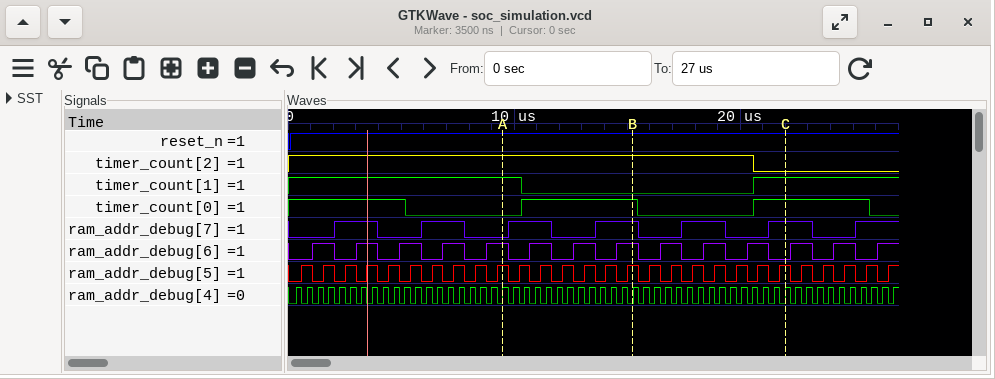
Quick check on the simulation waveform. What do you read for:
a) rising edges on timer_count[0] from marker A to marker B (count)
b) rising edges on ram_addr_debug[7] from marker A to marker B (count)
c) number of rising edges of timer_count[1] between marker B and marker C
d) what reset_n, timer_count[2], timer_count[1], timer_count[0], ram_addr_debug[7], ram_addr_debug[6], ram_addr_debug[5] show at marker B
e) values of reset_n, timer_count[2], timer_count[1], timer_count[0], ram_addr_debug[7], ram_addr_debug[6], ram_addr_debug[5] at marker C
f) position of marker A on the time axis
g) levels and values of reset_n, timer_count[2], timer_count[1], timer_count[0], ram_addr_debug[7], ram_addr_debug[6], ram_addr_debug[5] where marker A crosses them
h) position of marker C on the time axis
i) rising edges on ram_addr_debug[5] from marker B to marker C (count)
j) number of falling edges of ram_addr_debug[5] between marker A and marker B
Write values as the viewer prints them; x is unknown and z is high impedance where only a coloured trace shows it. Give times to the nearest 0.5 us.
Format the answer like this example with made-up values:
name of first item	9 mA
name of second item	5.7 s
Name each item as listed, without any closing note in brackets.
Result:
rising edges on timer_count[0] from marker A to marker B	1
rising edges on ram_addr_debug[7] from marker A to marker B	2
number of rising edges of timer_count[1] between marker B and marker C	1
what reset_n, timer_count[2], timer_count[1], timer_count[0], ram_addr_debug[7], ram_addr_debug[6], ram_addr_debug[5] show at marker B	reset_n=1, timer_count[2]=1, timer_count[1]=0, timer_count[0]=1, ram_addr_debug[7]=1, ram_addr_debug[6]=1, ram_addr_debug[5]=1
values of reset_n, timer_count[2], timer_count[1], timer_count[0], ram_addr_debug[7], ram_addr_debug[6], ram_addr_debug[5] at marker C	reset_n=1, timer_count[2]=0, timer_count[1]=1, timer_count[0]=1, ram_addr_debug[7]=1, ram_addr_debug[6]=0, ram_addr_debug[5]=1
position of marker A on the time axis	9.5 us
levels and values of reset_n, timer_count[2], timer_count[1], timer_count[0], ram_addr_debug[7], ram_addr_debug[6], ram_addr_debug[5] where marker A crosses them	reset_n=1, timer_count[2]=1, timer_count[1]=1, timer_count[0]=0, ram_addr_debug[7]=0, ram_addr_debug[6]=1, ram_addr_debug[5]=1
position of marker C on the time axis	22 us
rising edges on ram_addr_debug[5] from marker B to marker C	7
number of falling edges of ram_addr_debug[5] between marker A and marker B	6
